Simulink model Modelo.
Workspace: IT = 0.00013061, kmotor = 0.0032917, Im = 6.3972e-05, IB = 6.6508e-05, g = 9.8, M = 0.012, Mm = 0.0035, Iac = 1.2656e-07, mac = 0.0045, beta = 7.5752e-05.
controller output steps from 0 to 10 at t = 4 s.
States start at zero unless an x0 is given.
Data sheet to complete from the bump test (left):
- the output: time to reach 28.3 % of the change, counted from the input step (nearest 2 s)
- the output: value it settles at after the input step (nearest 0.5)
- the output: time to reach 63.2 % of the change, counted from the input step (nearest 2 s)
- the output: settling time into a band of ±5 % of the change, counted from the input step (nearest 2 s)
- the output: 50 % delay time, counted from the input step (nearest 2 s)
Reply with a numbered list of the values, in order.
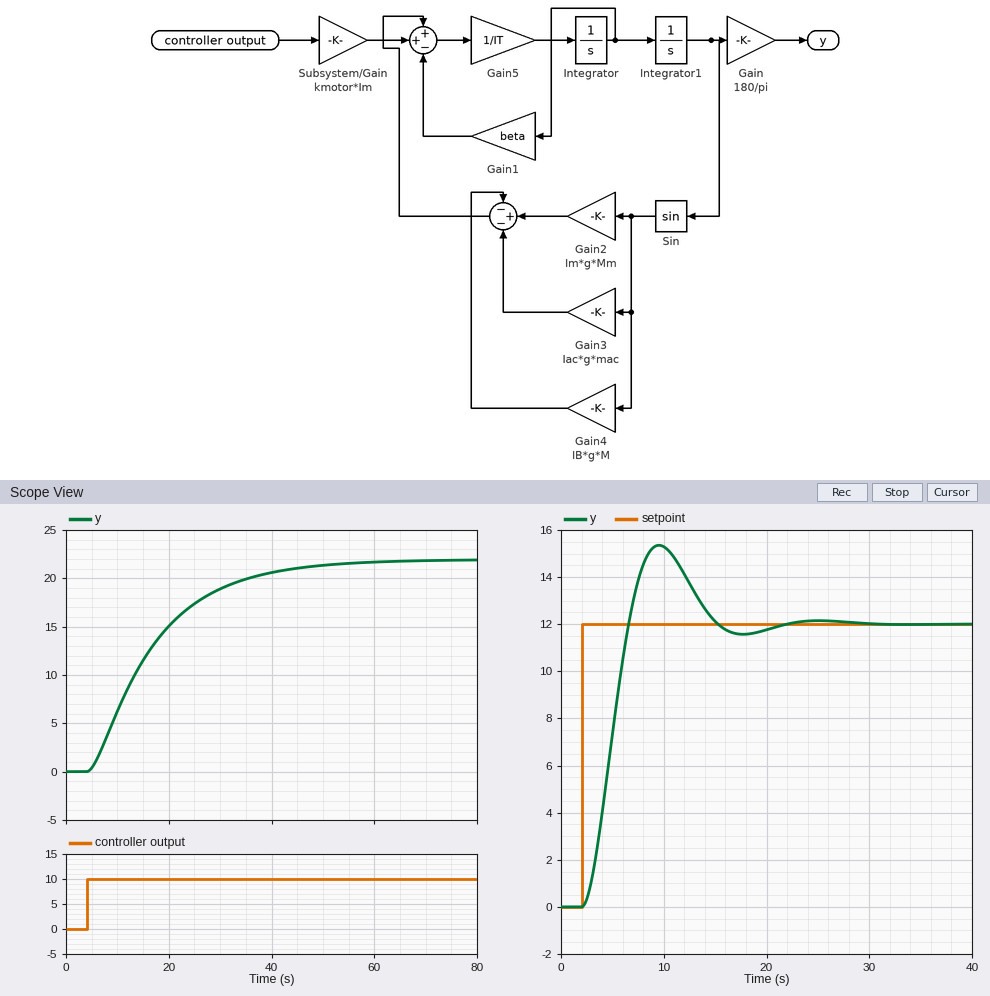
1. 6 s
2. 22.0
3. 14 s
4. 38 s
5. 10 s
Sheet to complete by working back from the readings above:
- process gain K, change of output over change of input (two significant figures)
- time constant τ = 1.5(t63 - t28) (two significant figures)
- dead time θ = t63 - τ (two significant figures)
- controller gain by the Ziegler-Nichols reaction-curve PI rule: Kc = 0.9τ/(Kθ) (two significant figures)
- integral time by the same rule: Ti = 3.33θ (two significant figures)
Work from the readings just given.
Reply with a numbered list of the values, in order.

1. 2.2
2. 12 s
3. 2.0 s
4. 2.5
5. 6.7 s
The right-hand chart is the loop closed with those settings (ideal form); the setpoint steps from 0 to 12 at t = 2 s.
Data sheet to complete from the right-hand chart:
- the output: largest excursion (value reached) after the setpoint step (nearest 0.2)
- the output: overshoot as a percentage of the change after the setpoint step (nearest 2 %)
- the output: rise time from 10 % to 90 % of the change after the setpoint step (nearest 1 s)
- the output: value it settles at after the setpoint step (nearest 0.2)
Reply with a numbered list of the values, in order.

1. 15.4
2. 28 %
3. 3 s
4. 12.0
